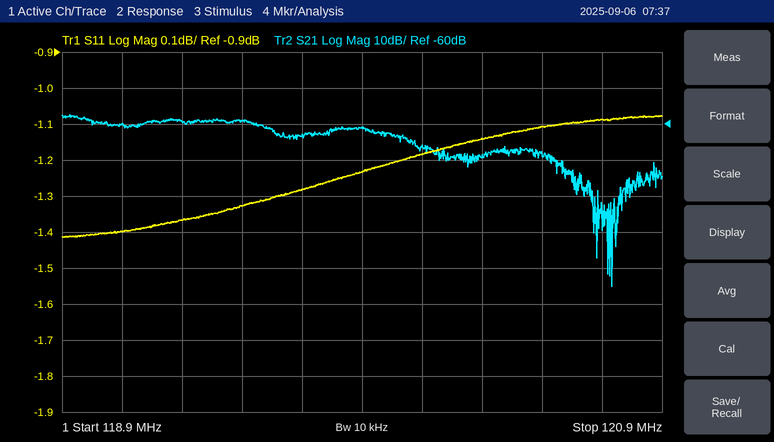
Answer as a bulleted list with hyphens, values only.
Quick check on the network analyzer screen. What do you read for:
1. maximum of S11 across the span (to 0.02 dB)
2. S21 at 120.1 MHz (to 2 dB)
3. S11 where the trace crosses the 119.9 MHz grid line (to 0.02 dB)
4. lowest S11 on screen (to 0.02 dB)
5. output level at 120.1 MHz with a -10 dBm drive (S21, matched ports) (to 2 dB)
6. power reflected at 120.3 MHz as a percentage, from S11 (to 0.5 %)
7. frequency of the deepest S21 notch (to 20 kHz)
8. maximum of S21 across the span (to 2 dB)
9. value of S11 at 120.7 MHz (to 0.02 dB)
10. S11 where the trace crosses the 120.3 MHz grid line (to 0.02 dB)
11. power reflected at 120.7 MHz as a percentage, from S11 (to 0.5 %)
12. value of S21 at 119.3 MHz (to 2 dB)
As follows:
- -1.08 dB
- -66 dB
- -1.24 dB
- -1.42 dB
- -76 dBm
- 77.0 %
- 120.74 MHz
- -58 dB
- -1.08 dB
- -1.14 dB
- 78.0 %
- -60 dB
